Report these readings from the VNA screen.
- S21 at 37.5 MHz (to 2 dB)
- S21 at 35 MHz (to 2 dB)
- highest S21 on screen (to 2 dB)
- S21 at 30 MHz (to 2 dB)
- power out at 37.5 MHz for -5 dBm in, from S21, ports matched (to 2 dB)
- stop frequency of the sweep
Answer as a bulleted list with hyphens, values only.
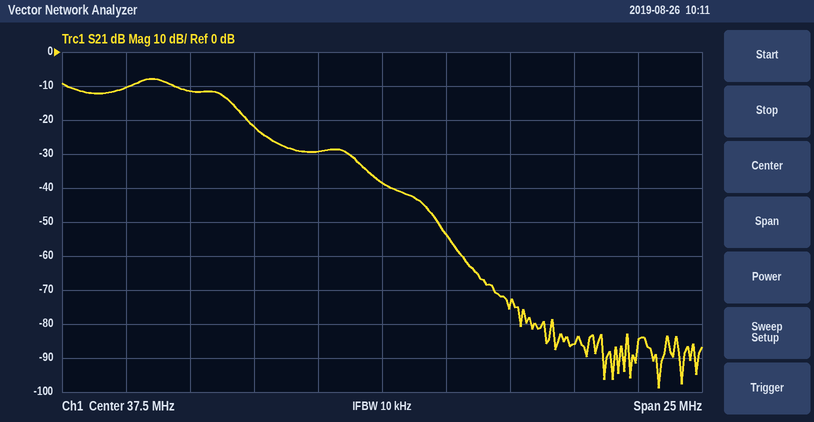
- -38 dB
- -30 dB
- -8 dB
- -12 dB
- -44 dBm
- 50 MHz
